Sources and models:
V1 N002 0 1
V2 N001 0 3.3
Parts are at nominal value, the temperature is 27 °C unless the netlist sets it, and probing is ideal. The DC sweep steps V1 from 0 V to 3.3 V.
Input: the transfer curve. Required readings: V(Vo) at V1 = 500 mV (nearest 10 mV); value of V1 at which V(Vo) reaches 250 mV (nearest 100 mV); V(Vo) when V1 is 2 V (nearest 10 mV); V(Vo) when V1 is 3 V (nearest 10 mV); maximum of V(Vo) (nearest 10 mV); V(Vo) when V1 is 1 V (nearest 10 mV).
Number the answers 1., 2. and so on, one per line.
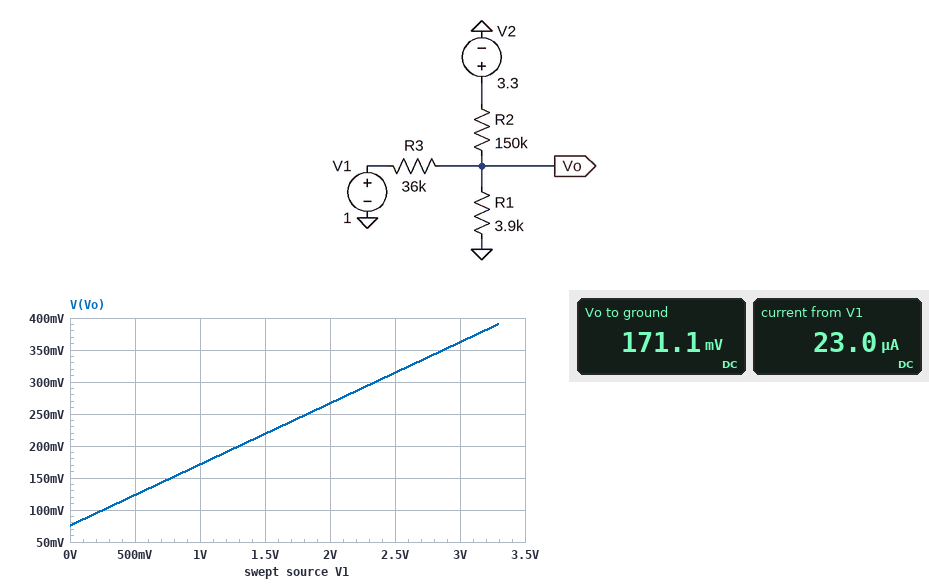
1. 120 mV
2. 1.8 V
3. 270 mV
4. 360 mV
5. 390 mV
6. 170 mV
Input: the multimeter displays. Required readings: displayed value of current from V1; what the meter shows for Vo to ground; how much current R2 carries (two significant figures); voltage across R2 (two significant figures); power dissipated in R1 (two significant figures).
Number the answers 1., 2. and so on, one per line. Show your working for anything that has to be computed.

1. 23.0 µA
2. 171.1 mV
3. (3.3 V - 171.1 mV) / 150 kΩ = 21 µA
4. 3.3 V - 171.1 mV = 3.1 V
5. (171.1 mV)^2 / 3.9 kΩ = 7.5 µW
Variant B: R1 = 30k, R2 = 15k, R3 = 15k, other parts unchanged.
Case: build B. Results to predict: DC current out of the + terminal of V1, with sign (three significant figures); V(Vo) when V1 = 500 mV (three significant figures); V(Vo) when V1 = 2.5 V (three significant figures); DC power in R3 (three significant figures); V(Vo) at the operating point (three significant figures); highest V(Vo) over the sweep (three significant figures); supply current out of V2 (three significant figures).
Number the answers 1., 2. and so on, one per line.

1. -48.0 µA
2. 1.52 V
3. 2.32 V
4. 34.6 µW
5. 1.72 V
6. 2.64 V
7. 105 µA
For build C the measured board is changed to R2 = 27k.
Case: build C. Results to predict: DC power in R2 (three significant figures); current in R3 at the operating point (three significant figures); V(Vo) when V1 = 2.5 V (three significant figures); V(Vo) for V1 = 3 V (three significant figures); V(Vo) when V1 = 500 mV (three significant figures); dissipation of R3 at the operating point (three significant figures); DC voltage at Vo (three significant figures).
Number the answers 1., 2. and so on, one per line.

1. 297 µW
2. 14.8 µA
3. 597 mV
4. 640 mV
5. 424 mV
6. 7.89 µW
7. 467 mV
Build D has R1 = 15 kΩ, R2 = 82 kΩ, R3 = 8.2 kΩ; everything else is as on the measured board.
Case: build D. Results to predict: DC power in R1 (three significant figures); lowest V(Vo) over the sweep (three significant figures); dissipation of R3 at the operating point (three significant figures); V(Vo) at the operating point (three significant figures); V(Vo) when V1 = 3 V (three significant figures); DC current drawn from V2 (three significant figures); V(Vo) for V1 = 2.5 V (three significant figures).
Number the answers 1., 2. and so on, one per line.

1. 43.5 µW
2. 200 mV
3. 4.51 µW
4. 808 mV
5. 2.02 V
6. 30.4 µA
7. 1.72 V
